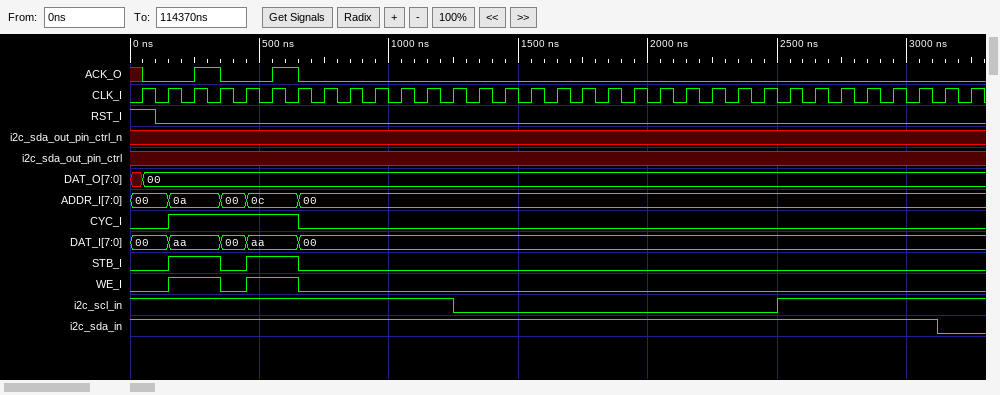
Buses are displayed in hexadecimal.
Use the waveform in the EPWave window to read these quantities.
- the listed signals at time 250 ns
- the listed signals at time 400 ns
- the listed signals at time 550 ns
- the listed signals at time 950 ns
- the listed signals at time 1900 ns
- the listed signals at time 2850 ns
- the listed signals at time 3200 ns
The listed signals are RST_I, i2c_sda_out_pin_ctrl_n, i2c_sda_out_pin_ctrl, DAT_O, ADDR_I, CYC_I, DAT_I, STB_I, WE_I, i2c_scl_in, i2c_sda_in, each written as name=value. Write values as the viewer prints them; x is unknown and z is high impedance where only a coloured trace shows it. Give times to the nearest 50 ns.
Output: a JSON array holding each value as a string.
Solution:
["RST_I=0, i2c_sda_out_pin_ctrl_n=x, i2c_sda_out_pin_ctrl=x, DAT_O=00, ADDR_I=0a, CYC_I=1, DAT_I=aa, STB_I=1, WE_I=1, i2c_scl_in=1, i2c_sda_in=1", "RST_I=0, i2c_sda_out_pin_ctrl_n=x, i2c_sda_out_pin_ctrl=x, DAT_O=00, ADDR_I=00, CYC_I=1, DAT_I=00, STB_I=0, WE_I=0, i2c_scl_in=1, i2c_sda_in=1", "RST_I=0, i2c_sda_out_pin_ctrl_n=x, i2c_sda_out_pin_ctrl=x, DAT_O=00, ADDR_I=0c, CYC_I=1, DAT_I=aa, STB_I=1, WE_I=1, i2c_scl_in=1, i2c_sda_in=1", "RST_I=0, i2c_sda_out_pin_ctrl_n=x, i2c_sda_out_pin_ctrl=x, DAT_O=00, ADDR_I=00, CYC_I=0, DAT_I=00, STB_I=0, WE_I=0, i2c_scl_in=1, i2c_sda_in=1", "RST_I=0, i2c_sda_out_pin_ctrl_n=x, i2c_sda_out_pin_ctrl=x, DAT_O=00, ADDR_I=00, CYC_I=0, DAT_I=00, STB_I=0, WE_I=0, i2c_scl_in=0, i2c_sda_in=1", "RST_I=0, i2c_sda_out_pin_ctrl_n=x, i2c_sda_out_pin_ctrl=x, DAT_O=00, ADDR_I=00, CYC_I=0, DAT_I=00, STB_I=0, WE_I=0, i2c_scl_in=1, i2c_sda_in=1", "RST_I=0, i2c_sda_out_pin_ctrl_n=x, i2c_sda_out_pin_ctrl=x, DAT_O=00, ADDR_I=00, CYC_I=0, DAT_I=00, STB_I=0, WE_I=0, i2c_scl_in=1, i2c_sda_in=0"]
